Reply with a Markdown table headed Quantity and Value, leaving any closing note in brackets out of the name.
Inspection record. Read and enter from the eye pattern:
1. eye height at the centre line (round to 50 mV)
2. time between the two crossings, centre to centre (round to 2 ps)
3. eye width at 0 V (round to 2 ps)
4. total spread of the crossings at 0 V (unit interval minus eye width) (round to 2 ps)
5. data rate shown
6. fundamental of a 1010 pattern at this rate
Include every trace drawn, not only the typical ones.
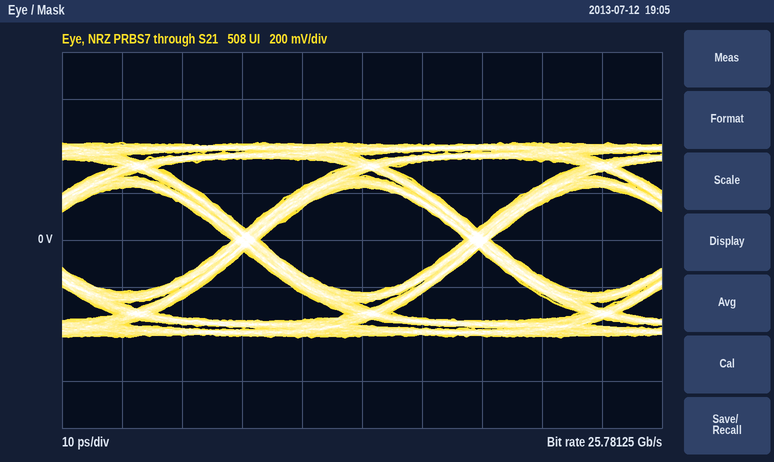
| Quantity | Value |
|---|---|
| eye height at the centre line | 450 mV |
| time between the two crossings, centre to centre | 38 ps |
| eye width at 0 V | 34 ps |
| total spread of the crossings at 0 V (unit interval minus eye width) | 4 ps |
| data rate shown | 25.78125 Gb/s |
| fundamental of a 1010 pattern at this rate | 12.89062 GHz |
